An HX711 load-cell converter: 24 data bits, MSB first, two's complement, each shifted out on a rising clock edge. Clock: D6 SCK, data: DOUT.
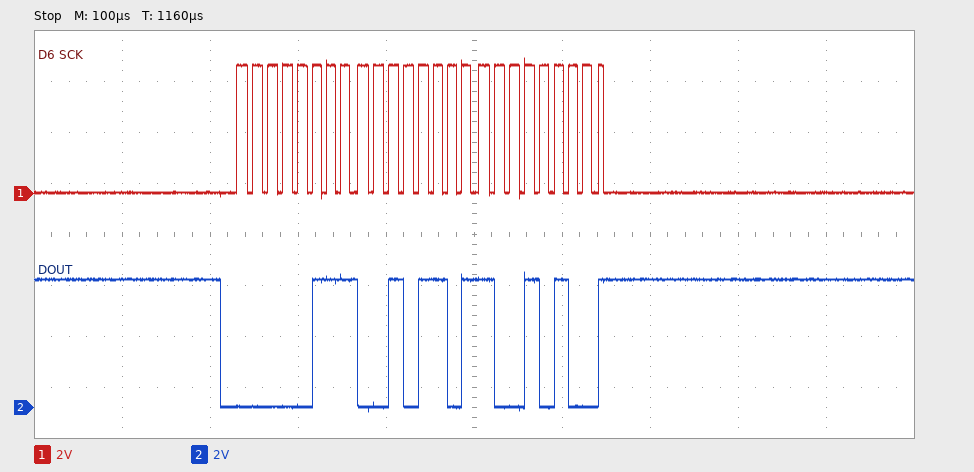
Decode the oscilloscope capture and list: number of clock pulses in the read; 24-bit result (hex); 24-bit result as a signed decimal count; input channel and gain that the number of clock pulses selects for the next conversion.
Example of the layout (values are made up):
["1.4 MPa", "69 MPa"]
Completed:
["25", "0x072D94", "470420", "channel A, gain 128"]
